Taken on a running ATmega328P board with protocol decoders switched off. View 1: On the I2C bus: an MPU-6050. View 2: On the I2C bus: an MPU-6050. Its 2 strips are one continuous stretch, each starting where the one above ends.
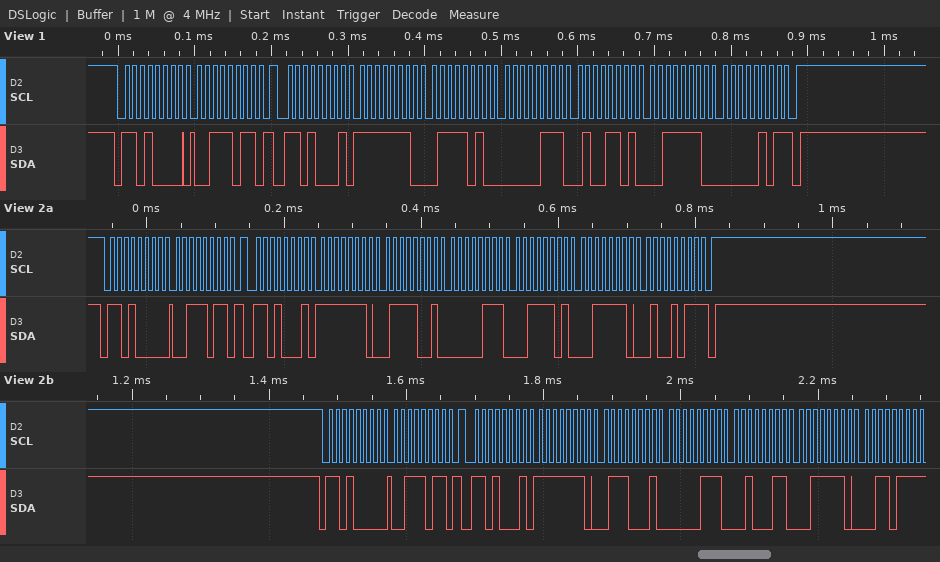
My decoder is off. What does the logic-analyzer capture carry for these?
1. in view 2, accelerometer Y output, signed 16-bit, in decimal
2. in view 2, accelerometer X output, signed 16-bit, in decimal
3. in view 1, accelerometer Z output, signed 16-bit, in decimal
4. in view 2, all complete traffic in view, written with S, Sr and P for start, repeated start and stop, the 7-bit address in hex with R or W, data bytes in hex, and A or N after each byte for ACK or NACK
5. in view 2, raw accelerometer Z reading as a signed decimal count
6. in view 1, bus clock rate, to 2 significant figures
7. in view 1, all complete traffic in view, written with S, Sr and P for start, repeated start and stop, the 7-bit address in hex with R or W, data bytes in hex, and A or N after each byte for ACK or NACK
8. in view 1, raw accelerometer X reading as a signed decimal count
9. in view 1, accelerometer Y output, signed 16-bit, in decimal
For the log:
1853
-391
15877
S 68W A 3B A Sr 68R A FE A 79 A 07 A 3D A 3E A 4B N P S 68W A 3B A Sr 68R A FE A 71 A 07 A 23 A 3E A 37 N
15947
100 kHz
S 68W A 3B A Sr 68R A FE A 7A A 07 A 4D A 3E A 05 N P
-390
1869
